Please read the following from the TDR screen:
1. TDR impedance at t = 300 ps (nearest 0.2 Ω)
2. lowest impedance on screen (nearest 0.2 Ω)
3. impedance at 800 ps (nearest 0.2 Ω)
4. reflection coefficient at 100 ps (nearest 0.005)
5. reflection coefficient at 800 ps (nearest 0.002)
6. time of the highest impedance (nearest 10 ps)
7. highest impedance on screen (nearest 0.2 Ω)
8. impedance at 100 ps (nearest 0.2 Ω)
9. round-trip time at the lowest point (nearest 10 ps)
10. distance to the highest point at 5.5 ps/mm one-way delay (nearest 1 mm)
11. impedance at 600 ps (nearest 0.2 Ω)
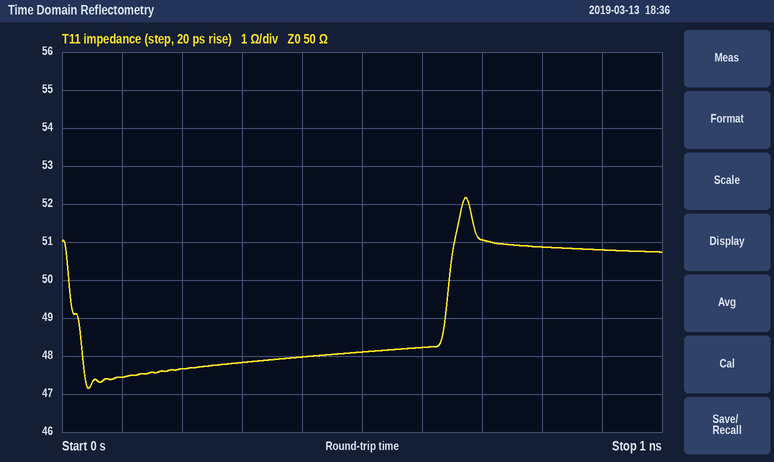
47.8 Ω
47.2 Ω
50.8 Ω
-0.025
+0.008
670 ps
52.2 Ω
47.4 Ω
40 ps
61 mm
48.2 Ω
